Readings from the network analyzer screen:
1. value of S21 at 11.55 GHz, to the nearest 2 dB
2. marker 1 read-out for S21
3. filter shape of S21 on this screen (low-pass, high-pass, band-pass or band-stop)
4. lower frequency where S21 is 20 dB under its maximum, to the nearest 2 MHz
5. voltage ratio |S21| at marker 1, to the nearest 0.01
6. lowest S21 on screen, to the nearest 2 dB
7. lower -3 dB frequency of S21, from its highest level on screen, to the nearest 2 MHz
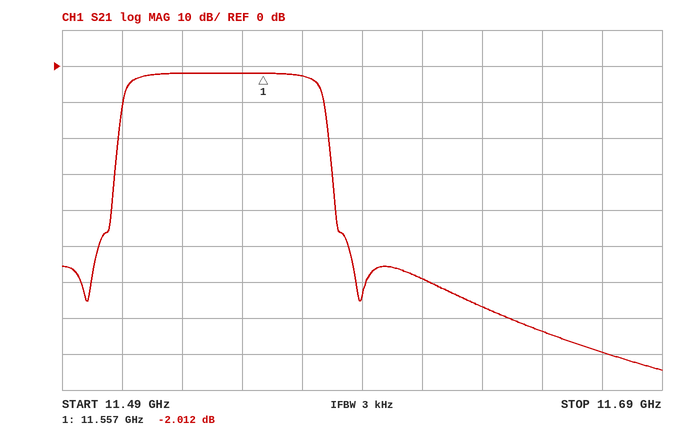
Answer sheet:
-2 dB
-2.012 dB
band-pass
11.508 GHz
0.79
-84 dB
11.512 GHz
